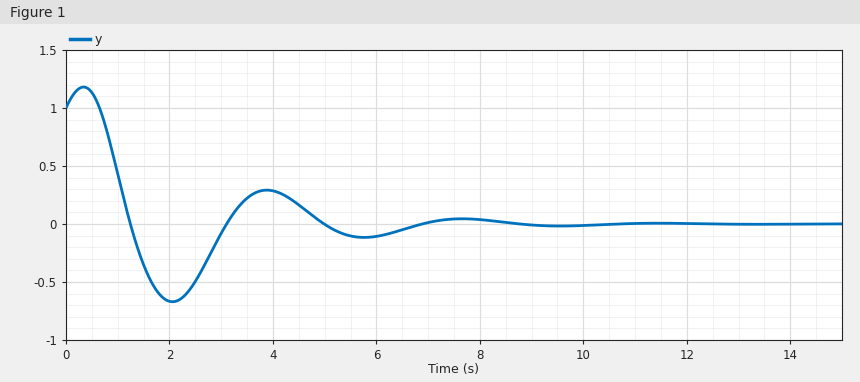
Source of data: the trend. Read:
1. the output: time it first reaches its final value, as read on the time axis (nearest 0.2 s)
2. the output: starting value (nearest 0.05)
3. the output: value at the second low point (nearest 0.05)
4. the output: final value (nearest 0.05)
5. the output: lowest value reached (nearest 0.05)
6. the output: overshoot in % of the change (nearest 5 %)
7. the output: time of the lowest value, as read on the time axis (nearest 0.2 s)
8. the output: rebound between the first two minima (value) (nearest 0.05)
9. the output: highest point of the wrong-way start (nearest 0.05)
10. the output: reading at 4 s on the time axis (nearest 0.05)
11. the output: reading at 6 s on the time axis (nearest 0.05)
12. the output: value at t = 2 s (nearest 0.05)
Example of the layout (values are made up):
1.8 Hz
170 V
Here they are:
1.2 s
1.00
-0.10
0.00
-0.65
65 %
2.0 s
0.30
1.20
0.30
-0.10
-0.65
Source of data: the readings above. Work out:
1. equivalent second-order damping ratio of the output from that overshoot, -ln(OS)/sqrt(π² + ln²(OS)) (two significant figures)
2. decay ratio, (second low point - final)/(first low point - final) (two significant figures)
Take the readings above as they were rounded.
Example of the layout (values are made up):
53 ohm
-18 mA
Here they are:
0.14
0.15
